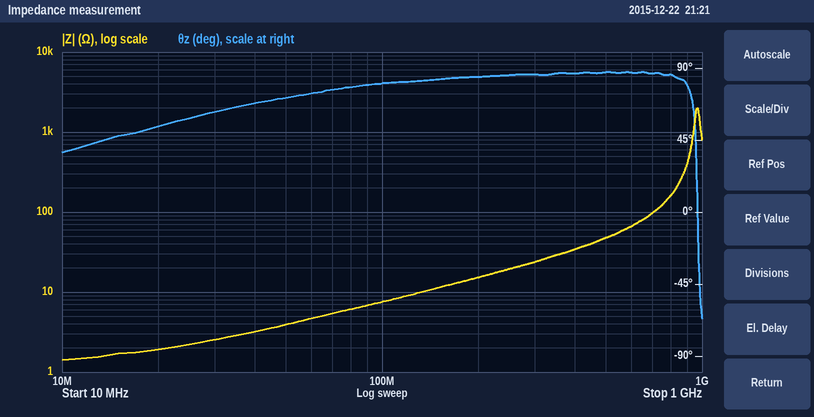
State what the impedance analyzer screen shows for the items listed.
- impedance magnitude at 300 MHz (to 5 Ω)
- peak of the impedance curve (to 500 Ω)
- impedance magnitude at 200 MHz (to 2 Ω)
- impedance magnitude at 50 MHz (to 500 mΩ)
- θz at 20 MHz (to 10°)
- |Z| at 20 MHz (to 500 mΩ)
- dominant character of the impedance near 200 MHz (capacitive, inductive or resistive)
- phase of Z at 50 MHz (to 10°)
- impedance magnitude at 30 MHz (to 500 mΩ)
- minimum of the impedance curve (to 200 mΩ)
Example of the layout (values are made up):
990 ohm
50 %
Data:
25 Ω
2.0 kΩ
16 Ω
4.0 Ω
50°
2.0 Ω
inductive
70°
2.5 Ω
1.4 Ω
